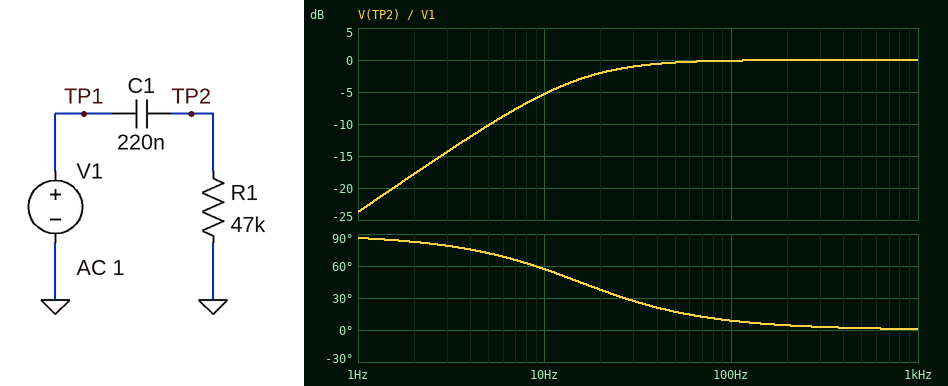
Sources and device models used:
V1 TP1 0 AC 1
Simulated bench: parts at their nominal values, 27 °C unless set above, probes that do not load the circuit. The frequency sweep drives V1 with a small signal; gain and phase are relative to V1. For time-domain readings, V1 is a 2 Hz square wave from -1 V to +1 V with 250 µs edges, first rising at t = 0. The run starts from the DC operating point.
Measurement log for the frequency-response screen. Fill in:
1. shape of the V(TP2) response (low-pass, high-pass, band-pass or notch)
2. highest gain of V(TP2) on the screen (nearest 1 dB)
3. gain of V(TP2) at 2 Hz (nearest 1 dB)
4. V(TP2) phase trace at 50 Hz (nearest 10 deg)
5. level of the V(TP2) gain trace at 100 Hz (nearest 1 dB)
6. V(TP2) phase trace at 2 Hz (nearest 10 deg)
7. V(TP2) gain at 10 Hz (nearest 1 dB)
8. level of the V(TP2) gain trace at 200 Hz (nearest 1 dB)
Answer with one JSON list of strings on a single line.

["high-pass", "0 dB", "-18 dB", "20 deg", "0 dB", "80 deg", "-5 dB", "0 dB"]
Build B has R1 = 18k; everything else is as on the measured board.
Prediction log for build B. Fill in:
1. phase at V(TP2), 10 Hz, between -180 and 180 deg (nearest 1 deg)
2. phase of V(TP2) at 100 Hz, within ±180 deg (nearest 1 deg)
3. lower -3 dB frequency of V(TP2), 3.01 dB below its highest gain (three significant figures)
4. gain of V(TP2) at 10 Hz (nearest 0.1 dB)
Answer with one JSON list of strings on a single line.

["76 deg", "22 deg", "40.2 Hz", "-12.3 dB"]
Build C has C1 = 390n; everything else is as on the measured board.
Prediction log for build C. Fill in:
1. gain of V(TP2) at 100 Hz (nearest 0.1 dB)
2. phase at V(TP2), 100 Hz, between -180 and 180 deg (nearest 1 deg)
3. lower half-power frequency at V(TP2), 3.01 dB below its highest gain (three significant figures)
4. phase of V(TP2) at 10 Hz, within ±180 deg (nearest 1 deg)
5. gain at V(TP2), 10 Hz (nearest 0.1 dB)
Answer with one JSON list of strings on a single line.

["0 dB", "5 deg", "8.68 Hz", "41 deg", "-2.4 dB"]
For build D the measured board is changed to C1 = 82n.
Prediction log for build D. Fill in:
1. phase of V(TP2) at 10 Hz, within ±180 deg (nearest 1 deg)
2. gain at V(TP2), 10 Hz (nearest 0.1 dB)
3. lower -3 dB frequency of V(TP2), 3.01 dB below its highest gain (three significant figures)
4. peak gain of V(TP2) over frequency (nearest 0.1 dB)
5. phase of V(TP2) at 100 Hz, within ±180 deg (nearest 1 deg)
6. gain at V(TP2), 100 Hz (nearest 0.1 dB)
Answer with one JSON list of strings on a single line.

["76 deg", "-12.6 dB", "41.3 Hz", "0 dB", "22 deg", "-0.7 dB"]
